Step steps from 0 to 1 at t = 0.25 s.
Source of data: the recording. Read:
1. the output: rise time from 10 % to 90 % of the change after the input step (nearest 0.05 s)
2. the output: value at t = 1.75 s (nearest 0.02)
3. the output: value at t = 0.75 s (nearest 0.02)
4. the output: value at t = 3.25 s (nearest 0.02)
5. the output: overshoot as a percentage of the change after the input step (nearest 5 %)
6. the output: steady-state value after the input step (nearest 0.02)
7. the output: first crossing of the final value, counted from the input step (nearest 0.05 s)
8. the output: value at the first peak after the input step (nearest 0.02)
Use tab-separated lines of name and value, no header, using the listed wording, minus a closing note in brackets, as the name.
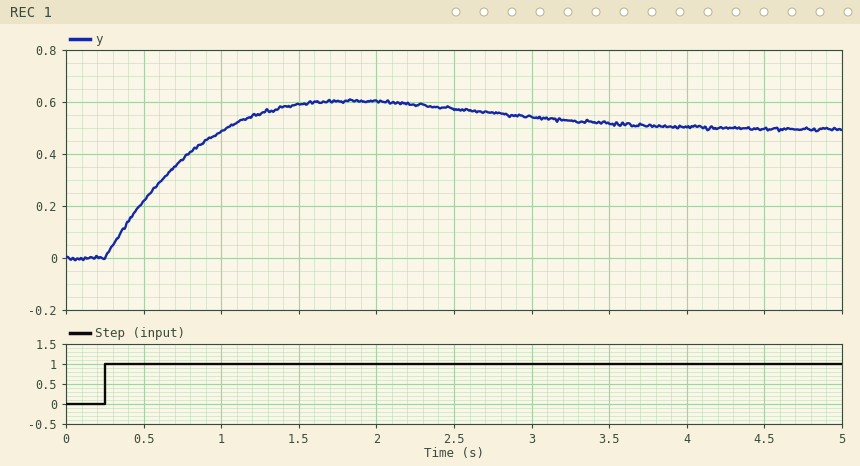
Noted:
the output: rise time from 10 % to 90 % of the change after the input step	0.60 s
the output: value at t = 1.75 s	0.60
the output: value at t = 0.75 s	0.38
the output: value at t = 3.25 s	0.52
the output: overshoot as a percentage of the change after the input step	20 %
the output: steady-state value after the input step	0.50
the output: first crossing of the final value, counted from the input step	0.80 s
the output: value at the first peak after the input step	0.60
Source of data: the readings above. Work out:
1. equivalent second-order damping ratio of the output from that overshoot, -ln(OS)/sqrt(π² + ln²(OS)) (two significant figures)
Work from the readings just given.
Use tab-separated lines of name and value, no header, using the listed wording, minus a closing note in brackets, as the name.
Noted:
equivalent second-order damping ratio of the output from that overshoot, -ln(OS)/sqrt(π² + ln²(OS))	0.46
